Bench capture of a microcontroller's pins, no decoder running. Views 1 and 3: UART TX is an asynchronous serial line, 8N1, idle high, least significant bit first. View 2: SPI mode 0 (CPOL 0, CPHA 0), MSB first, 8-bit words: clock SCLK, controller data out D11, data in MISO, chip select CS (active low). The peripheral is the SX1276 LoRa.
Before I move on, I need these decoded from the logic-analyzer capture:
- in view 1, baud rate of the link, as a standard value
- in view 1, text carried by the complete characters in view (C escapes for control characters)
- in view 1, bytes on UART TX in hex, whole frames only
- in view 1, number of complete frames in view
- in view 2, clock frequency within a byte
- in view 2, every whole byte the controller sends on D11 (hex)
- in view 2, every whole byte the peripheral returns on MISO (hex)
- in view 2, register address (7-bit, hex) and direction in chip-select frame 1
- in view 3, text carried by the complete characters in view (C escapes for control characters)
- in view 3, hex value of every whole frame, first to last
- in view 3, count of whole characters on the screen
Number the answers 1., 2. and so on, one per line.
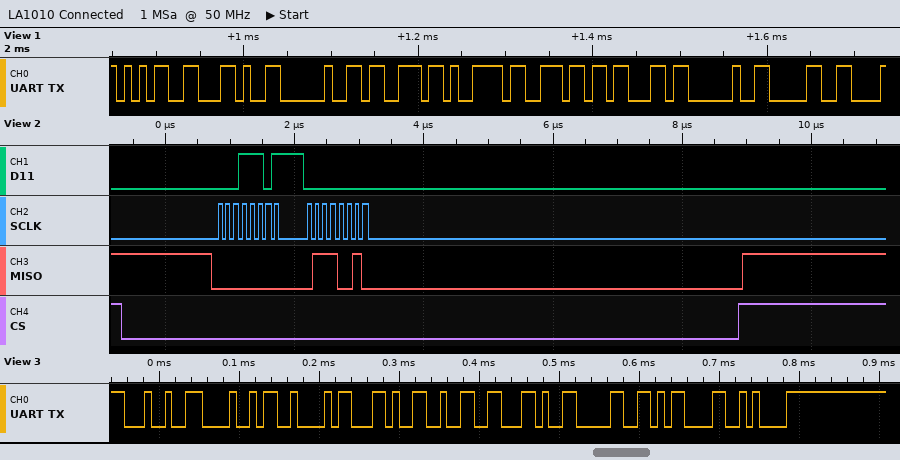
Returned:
1. 115200 baud
2. "5, sync 0"
3. 0x35 0x2C 0x20 0x73 0x79 0x6E 0x63 0x20 0x30
4. 9
5. 8 MHz
6. 1D 00
7. 00 72
8. 0x1D read
9. "$HB,2,0\r\n"
10. 0x24 0x48 0x42 0x2C 0x32 0x2C 0x30 0x0D 0x0A
11. 9
